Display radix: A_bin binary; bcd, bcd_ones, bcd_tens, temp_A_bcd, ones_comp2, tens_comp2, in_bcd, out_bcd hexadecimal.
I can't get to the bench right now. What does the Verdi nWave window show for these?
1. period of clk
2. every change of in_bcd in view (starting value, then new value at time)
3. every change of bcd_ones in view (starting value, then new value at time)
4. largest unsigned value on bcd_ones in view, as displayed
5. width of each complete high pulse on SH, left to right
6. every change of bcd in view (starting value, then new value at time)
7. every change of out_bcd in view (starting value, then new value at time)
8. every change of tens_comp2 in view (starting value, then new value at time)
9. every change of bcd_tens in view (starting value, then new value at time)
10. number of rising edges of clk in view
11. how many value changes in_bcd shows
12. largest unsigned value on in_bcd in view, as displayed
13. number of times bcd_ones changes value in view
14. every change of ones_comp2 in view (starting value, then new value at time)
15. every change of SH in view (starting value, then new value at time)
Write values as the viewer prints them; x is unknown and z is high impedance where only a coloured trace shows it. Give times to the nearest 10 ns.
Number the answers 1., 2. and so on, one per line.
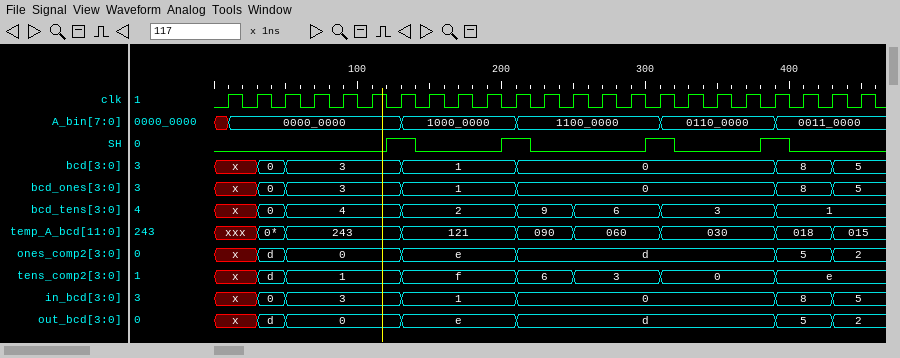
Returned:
1. 20 ns
2. x, 0 at 30 ns, 3 at 50 ns, 1 at 130 ns, 0 at 210 ns, 8 at 390 ns, 5 at 430 ns
3. x, 0 at 30 ns, 3 at 50 ns, 1 at 130 ns, 0 at 210 ns, 8 at 390 ns, 5 at 430 ns
4. 8
5. 20 ns, 20 ns, 20 ns, 20 ns
6. x, 0 at 30 ns, 3 at 50 ns, 1 at 130 ns, 0 at 210 ns, 8 at 390 ns, 5 at 430 ns
7. x, d at 30 ns, 0 at 50 ns, e at 130 ns, d at 210 ns, 5 at 390 ns, 2 at 430 ns
8. x, d at 30 ns, 1 at 50 ns, f at 130 ns, 6 at 210 ns, 3 at 250 ns, 0 at 310 ns, e at 390 ns
9. x, 0 at 30 ns, 4 at 50 ns, 2 at 130 ns, 9 at 210 ns, 6 at 250 ns, 3 at 310 ns, 1 at 390 ns
10. 23
11. 6
12. 8
13. 6
14. x, d at 30 ns, 0 at 50 ns, e at 130 ns, d at 210 ns, 5 at 390 ns, 2 at 430 ns
15. 0, 1 at 120 ns, 0 at 140 ns, 1 at 200 ns, 0 at 220 ns, 1 at 300 ns, 0 at 320 ns, 1 at 380 ns, 0 at 400 ns
